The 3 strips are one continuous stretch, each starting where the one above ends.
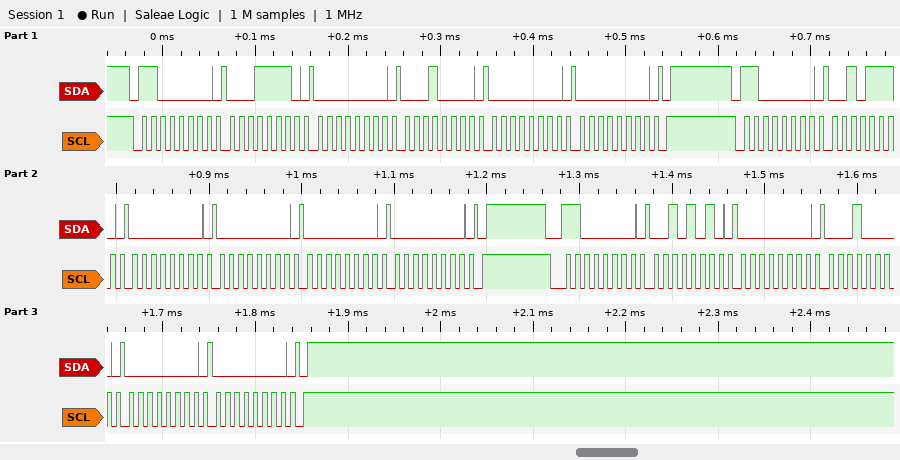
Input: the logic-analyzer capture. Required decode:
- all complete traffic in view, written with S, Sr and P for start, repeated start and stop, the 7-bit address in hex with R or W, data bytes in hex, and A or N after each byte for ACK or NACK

S 60W A 1E A 00 A 10 A 00 A 00 A P S 60W A 2E A 00 A 00 A 00 A 00 A P S 60W A 2A A 00 A 10 A 00 A 00 A P
